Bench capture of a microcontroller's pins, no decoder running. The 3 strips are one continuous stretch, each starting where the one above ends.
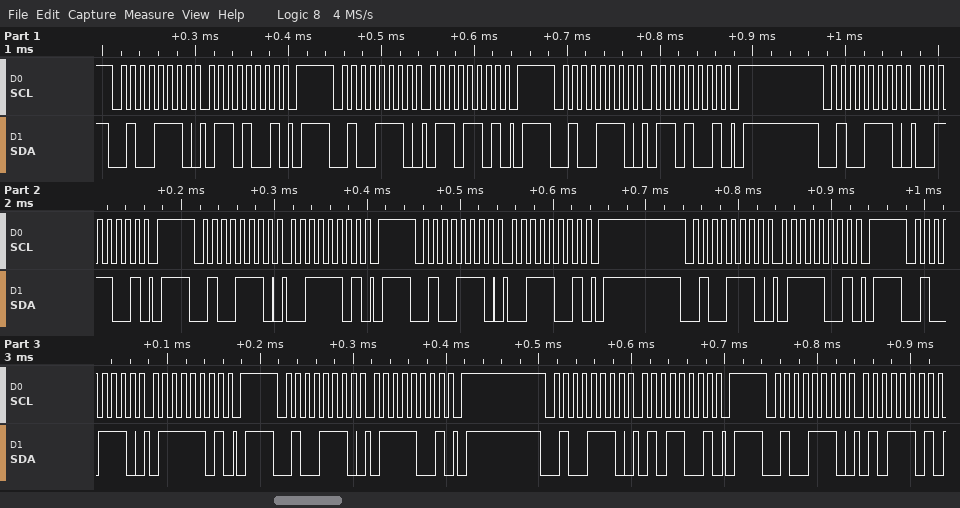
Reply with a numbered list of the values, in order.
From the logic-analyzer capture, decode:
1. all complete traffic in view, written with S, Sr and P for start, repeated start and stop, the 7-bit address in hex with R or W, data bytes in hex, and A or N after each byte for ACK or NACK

1. S 27W A 69 A P S 27W A 6D A P S 27W A 69 A P S 27W A 39 A P S 27W A 3D A P S 27W A 39 A P S 27W A 79 A P S 27W A 7D A P S 27W A 79 A P S 27W A 59 A P S 27W A 5D A
